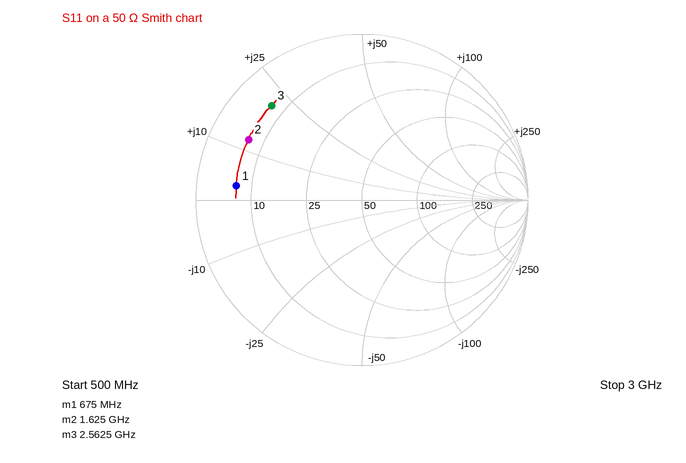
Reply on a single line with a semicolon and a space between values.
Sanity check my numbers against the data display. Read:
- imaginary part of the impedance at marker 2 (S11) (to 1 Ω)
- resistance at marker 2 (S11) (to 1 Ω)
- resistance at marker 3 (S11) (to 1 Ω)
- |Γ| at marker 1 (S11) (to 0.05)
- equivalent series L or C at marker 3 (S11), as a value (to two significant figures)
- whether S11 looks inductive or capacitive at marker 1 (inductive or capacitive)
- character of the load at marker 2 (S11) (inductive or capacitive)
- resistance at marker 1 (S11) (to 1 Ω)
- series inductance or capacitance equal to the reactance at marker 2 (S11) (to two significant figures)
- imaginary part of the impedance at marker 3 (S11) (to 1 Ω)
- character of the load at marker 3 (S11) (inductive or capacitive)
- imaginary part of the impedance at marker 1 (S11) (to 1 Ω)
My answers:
+12 Ω; 7 Ω; 7 Ω; 0.75; 1.3 nH; inductive; inductive; 7 Ω; 1.2 nH; +21 Ω; inductive; +3 Ω
